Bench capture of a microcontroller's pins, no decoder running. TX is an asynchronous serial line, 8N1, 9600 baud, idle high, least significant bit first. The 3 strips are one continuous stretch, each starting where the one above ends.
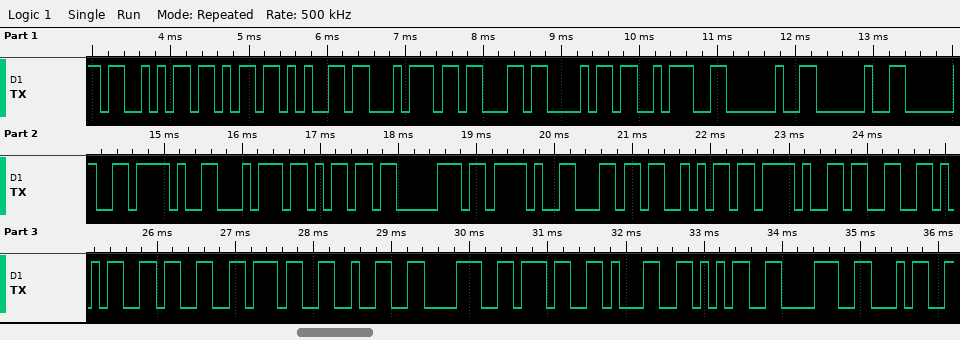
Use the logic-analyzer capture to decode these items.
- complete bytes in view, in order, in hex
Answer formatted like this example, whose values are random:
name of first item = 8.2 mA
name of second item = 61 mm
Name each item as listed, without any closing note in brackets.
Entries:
complete bytes in view, in order, in hex = 53 6B 65 74 63 68 3A 20 20 20 2F 74 6D 70 2F 6C 6A 2F 33 35 33 37 32 38 37 31 35 38 34
